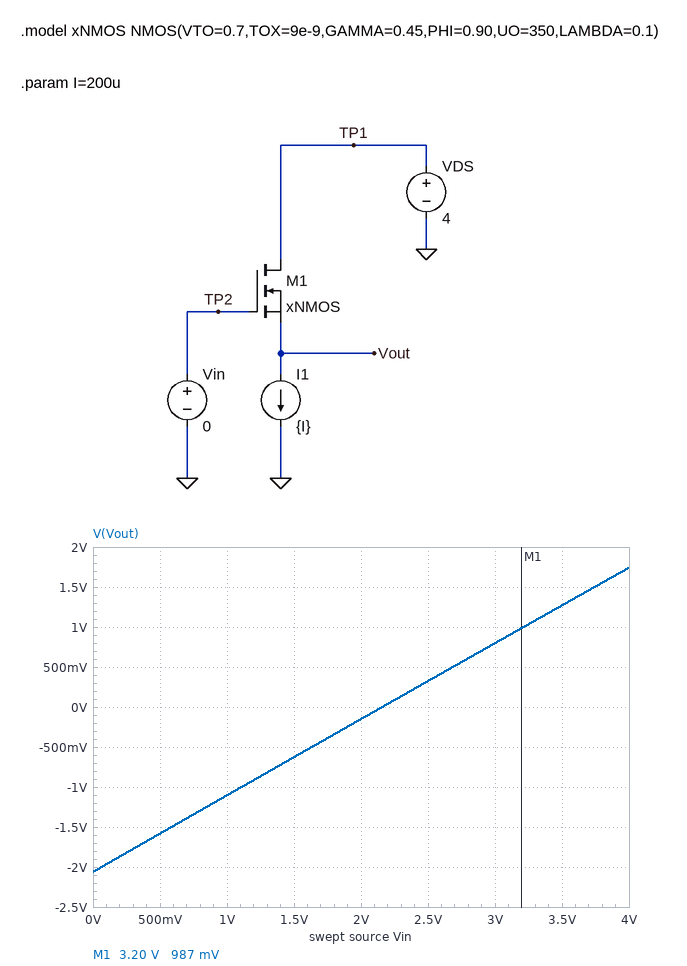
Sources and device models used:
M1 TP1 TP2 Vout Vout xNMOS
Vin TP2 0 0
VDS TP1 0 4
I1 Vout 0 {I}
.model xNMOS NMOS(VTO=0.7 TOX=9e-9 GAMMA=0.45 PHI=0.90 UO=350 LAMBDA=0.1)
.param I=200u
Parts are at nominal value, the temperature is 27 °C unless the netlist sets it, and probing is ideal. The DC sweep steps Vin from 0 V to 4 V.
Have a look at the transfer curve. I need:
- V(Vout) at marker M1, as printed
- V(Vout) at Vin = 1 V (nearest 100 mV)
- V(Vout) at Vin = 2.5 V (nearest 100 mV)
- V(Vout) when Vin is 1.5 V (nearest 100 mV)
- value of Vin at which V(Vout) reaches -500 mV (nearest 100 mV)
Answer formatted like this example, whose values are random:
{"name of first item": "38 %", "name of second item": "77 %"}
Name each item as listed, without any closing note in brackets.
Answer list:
{"V(Vout) at marker M1, as printed": "987 mV", "V(Vout) at Vin = 1 V": "-1.1 V", "V(Vout) at Vin = 2.5 V": "300 mV", "V(Vout) when Vin is 1.5 V": "-600 mV", "value of Vin at which V(Vout) reaches -500 mV": "1.6 V"}
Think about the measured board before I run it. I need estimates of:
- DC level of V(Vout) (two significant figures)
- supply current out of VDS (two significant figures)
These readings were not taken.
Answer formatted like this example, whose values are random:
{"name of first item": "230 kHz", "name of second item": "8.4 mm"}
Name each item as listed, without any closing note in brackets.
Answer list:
{"DC level of V(Vout)": "-2.1 V", "supply current out of VDS": "200 µA"}
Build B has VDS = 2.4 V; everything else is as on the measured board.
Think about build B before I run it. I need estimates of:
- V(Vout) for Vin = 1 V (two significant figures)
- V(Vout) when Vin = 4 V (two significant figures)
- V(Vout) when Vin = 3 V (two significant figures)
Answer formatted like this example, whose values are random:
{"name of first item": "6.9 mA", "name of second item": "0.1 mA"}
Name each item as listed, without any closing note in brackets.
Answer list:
{"V(Vout) for Vin = 1 V": "-1.2 V", "V(Vout) when Vin = 4 V": "1.4 V", "V(Vout) when Vin = 3 V": "700 mV"}
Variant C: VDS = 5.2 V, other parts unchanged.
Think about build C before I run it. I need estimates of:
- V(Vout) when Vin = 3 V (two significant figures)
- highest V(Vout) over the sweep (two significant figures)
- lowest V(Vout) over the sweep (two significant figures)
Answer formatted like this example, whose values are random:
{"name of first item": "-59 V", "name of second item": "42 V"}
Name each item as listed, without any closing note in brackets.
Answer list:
{"V(Vout) when Vin = 3 V": "860 mV", "highest V(Vout) over the sweep": "1.8 V", "lowest V(Vout) over the sweep": "-2.0 V"}
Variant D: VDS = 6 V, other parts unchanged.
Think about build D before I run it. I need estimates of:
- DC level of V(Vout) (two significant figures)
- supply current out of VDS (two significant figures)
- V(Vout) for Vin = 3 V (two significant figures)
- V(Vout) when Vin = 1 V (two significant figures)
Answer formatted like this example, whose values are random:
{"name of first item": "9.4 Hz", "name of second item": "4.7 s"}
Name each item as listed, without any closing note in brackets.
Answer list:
{"DC level of V(Vout)": "-2.0 V", "supply current out of VDS": "200 µA", "V(Vout) for Vin = 3 V": "900 mV", "V(Vout) when Vin = 1 V": "-1.0 V"}
